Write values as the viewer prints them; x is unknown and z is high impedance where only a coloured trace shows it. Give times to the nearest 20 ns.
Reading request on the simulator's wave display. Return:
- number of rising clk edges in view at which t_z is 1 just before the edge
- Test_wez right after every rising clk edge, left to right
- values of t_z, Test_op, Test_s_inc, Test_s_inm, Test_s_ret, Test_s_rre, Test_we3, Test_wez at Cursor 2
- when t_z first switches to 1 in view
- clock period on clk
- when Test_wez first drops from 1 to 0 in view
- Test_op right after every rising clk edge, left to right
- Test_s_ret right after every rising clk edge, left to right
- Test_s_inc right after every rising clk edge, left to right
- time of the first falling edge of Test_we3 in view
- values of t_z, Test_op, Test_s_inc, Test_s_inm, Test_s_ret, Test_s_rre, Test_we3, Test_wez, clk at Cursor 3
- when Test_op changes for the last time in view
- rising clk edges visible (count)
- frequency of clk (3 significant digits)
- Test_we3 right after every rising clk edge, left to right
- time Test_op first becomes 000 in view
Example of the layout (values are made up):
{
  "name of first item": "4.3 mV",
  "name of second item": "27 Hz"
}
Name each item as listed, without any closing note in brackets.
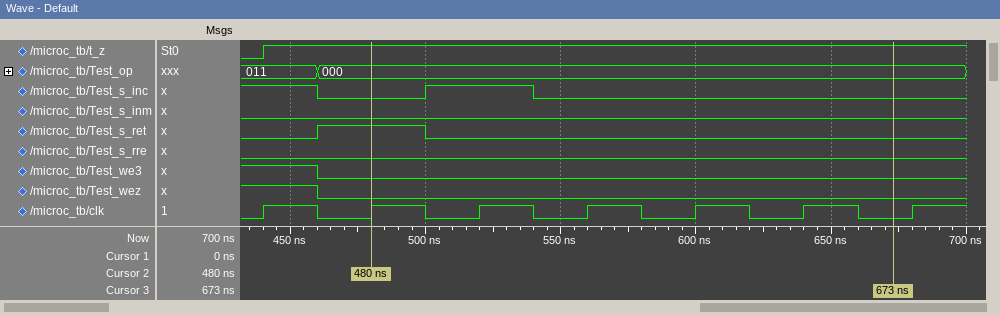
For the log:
{
  "number of rising clk edges in view at which t_z is 1 just before the edge": "6",
  "Test_wez right after every rising clk edge, left to right": "1 0 0 0 0 0 0",
  "values of t_z, Test_op, Test_s_inc, Test_s_inm, Test_s_ret, Test_s_rre, Test_we3, Test_wez at Cursor 2": "t_z=1, Test_op=000, Test_s_inc=0, Test_s_inm=0, Test_s_ret=1, Test_s_rre=0, Test_we3=0, Test_wez=0",
  "when t_z first switches to 1 in view": "440 ns",
  "clock period on clk": "40 ns",
  "when Test_wez first drops from 1 to 0 in view": "460 ns",
  "Test_op right after every rising clk edge, left to right": "011, 000, 000, 000, 000, 000, 000",
  "Test_s_ret right after every rising clk edge, left to right": "0 1 0 0 0 0 0",
  "Test_s_inc right after every rising clk edge, left to right": "1 0 1 0 0 0 0",
  "time of the first falling edge of Test_we3 in view": "460 ns",
  "values of t_z, Test_op, Test_s_inc, Test_s_inm, Test_s_ret, Test_s_rre, Test_we3, Test_wez, clk at Cursor 3": "t_z=1, Test_op=000, Test_s_inc=0, Test_s_inm=0, Test_s_ret=0, Test_s_rre=0, Test_we3=0, Test_wez=0, clk=0",
  "when Test_op changes for the last time in view": "460 ns",
  "rising clk edges visible": "7",
  "frequency of clk": "25.0 MHz",
  "Test_we3 right after every rising clk edge, left to right": "1 0 0 0 0 0 0",
  "time Test_op first becomes 000 in view": "460 ns"
}
